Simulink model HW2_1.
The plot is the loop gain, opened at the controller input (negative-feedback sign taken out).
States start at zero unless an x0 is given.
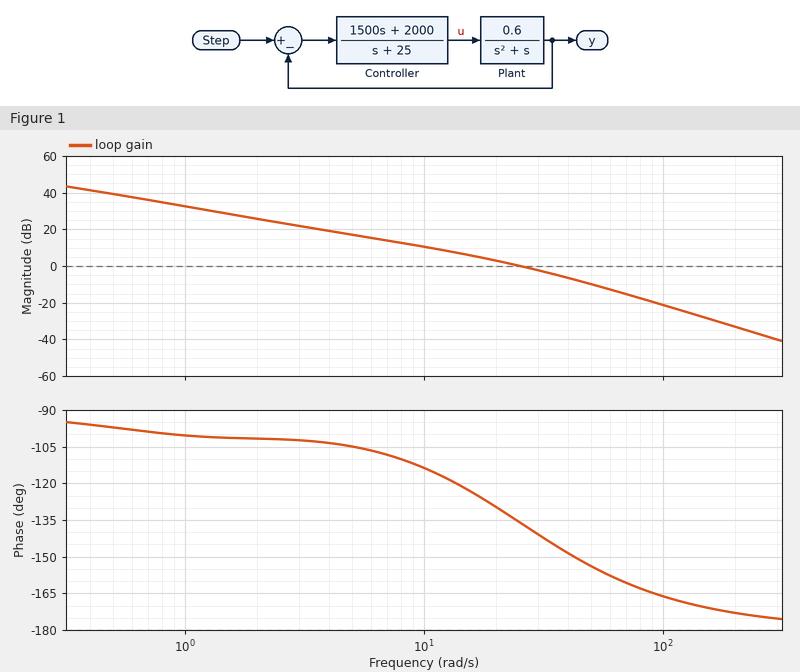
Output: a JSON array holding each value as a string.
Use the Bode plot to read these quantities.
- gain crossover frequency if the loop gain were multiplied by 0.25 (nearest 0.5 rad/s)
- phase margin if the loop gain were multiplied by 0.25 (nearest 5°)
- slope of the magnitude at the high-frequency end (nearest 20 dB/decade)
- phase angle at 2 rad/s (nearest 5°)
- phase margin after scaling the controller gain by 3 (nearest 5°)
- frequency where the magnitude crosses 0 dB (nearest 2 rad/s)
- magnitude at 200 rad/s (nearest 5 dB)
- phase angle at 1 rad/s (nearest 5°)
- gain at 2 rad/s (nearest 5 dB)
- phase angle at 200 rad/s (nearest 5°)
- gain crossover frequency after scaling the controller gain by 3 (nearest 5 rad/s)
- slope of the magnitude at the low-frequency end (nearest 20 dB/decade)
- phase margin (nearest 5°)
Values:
["8.5 rad/s", "70°", "-40 dB/decade", "-100°", "25°", "26 rad/s", "-35 dB", "-100°", "25 dB", "-175°", "50 rad/s", "-20 dB/decade", "45°"]
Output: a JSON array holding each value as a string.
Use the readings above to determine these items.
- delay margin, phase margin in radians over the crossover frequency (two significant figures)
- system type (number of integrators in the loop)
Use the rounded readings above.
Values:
["0.030 s", "1"]
